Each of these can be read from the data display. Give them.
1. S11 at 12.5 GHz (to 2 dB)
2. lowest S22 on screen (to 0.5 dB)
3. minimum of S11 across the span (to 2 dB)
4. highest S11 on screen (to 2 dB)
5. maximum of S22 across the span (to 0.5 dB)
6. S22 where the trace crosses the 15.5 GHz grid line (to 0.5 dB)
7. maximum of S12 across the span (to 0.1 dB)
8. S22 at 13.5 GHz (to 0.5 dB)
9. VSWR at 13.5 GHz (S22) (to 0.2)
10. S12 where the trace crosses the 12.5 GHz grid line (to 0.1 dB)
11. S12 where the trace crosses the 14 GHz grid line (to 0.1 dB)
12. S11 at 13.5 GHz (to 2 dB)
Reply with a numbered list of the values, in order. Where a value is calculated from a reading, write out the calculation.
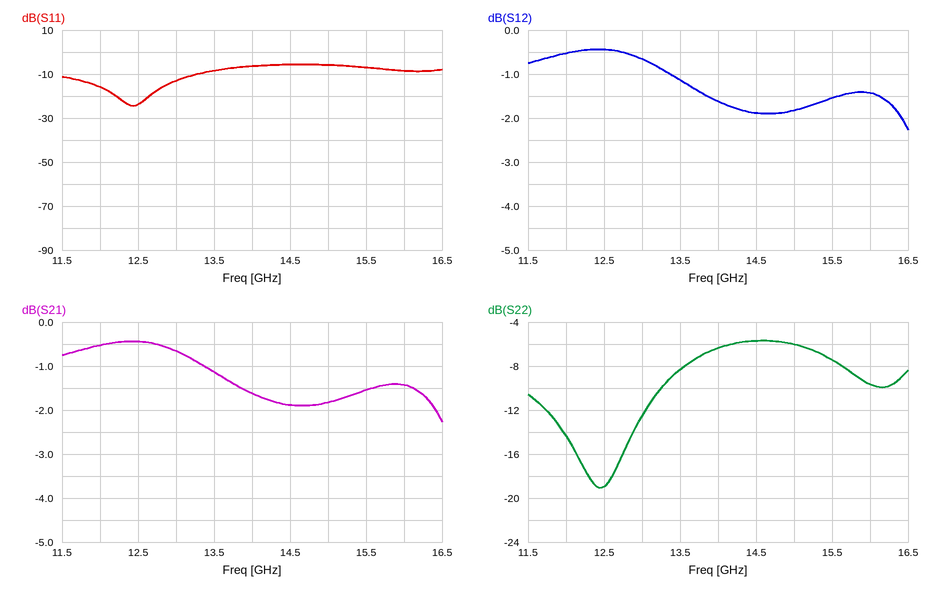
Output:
1. -24 dB
2. -19.0 dB
3. -24 dB
4. -6 dB
5. -5.5 dB
6. -7.5 dB
7. -0.4 dB
8. -8.5 dB
9. |Γ| = 10^(-8.5/20) = 0.3758; VSWR = (1 + 0.3758)/(1 − 0.3758) ≈ 2.2
10. -0.4 dB
11. -1.6 dB
12. -8 dB
